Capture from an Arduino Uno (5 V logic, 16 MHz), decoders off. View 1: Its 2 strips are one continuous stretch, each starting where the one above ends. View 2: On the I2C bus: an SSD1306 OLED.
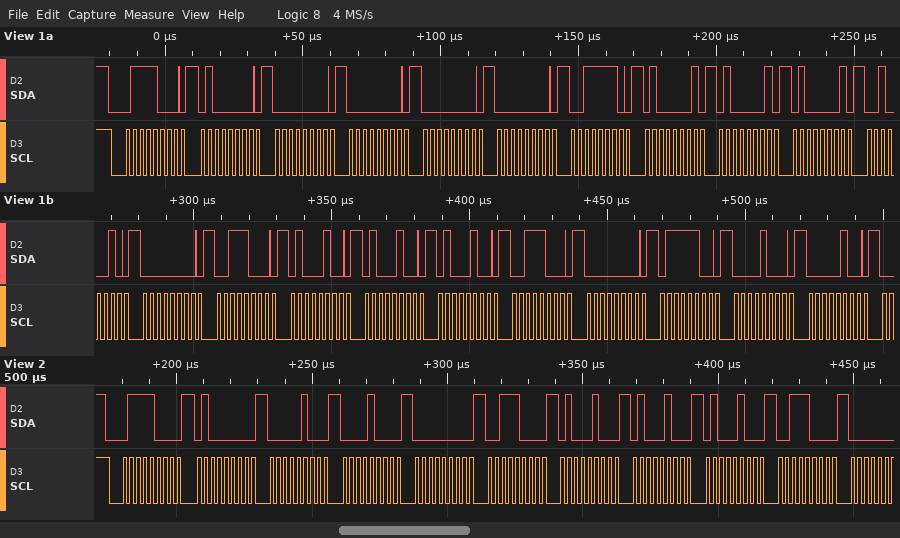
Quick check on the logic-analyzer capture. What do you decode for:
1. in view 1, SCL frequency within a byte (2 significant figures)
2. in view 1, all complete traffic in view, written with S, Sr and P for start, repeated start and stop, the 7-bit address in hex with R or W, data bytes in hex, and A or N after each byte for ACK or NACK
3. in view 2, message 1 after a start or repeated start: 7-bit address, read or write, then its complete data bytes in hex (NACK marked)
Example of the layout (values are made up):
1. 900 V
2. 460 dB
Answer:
1. 400 kHz
2. S 3CW A 40 A 00 A 00 A 00 A 00 A 3E A 41 A 41 A 41 A 22 A 00 A 38 A 44 A 44 A 44 A 38 A 00 A 7C A 08 A 04 A
3. 0x3C write: 40 04 08 00 38 44 44 44 38
